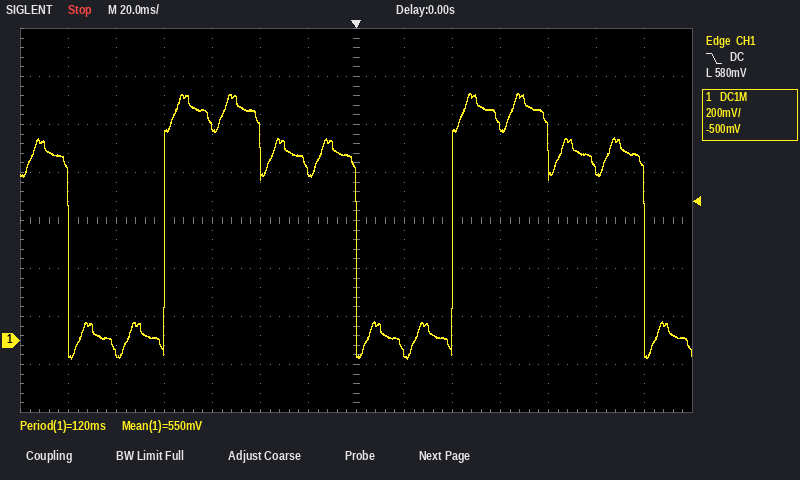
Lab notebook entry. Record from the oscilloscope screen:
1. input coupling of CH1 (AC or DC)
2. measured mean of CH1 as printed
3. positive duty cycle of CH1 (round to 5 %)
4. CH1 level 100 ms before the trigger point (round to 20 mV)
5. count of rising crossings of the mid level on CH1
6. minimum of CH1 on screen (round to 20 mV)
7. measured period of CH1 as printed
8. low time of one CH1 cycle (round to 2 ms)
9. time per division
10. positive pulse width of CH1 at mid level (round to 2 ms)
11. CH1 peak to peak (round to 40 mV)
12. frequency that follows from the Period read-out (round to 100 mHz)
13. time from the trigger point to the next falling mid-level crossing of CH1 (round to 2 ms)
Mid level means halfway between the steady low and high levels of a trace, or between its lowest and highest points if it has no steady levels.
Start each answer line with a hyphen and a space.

- DC
- 550 mV
- 65 %
- -60 mV
- 2
- -80 mV
- 120 ms
- 40 ms
- 20 ms
- 80 ms
- 1.12 V
- 8.3 Hz
- 120 ms
